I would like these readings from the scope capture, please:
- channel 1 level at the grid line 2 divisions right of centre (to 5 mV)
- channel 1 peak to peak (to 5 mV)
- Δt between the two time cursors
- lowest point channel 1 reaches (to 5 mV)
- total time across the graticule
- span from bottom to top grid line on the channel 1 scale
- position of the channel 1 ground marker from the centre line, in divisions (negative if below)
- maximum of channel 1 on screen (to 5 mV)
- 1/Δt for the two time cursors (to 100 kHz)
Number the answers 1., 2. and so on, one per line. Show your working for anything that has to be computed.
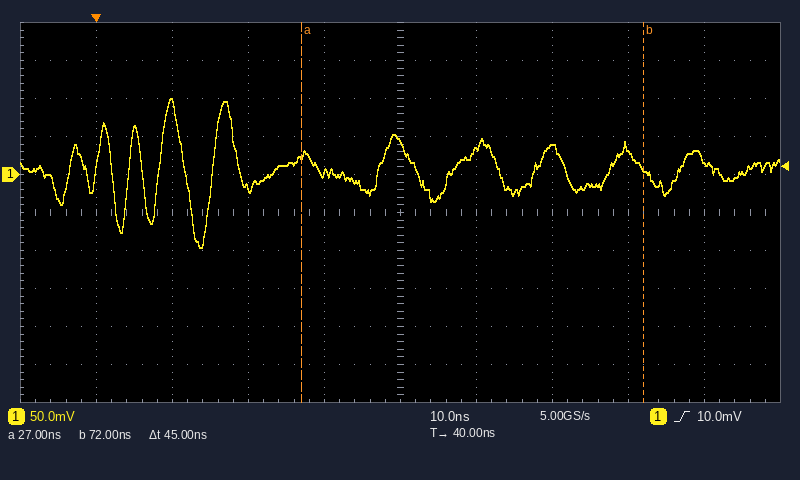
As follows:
1. 35 mV
2. 100 mV − (-95 mV) = 195 mV
3. 45 ns
4. -95 mV
5. 100 ns
6. 500 mV
7. +1.0 div
8. 100 mV
9. 1 / 45 ns ≈ 22.2 MHz
